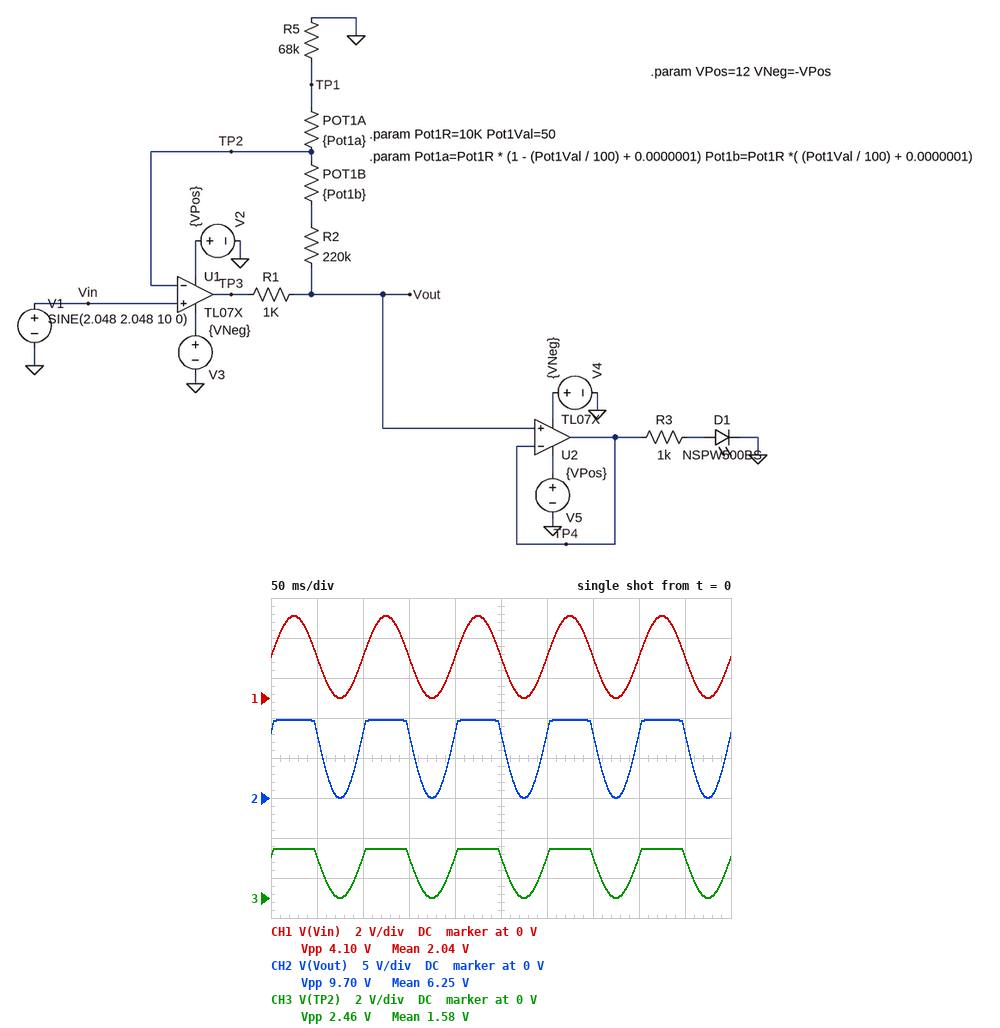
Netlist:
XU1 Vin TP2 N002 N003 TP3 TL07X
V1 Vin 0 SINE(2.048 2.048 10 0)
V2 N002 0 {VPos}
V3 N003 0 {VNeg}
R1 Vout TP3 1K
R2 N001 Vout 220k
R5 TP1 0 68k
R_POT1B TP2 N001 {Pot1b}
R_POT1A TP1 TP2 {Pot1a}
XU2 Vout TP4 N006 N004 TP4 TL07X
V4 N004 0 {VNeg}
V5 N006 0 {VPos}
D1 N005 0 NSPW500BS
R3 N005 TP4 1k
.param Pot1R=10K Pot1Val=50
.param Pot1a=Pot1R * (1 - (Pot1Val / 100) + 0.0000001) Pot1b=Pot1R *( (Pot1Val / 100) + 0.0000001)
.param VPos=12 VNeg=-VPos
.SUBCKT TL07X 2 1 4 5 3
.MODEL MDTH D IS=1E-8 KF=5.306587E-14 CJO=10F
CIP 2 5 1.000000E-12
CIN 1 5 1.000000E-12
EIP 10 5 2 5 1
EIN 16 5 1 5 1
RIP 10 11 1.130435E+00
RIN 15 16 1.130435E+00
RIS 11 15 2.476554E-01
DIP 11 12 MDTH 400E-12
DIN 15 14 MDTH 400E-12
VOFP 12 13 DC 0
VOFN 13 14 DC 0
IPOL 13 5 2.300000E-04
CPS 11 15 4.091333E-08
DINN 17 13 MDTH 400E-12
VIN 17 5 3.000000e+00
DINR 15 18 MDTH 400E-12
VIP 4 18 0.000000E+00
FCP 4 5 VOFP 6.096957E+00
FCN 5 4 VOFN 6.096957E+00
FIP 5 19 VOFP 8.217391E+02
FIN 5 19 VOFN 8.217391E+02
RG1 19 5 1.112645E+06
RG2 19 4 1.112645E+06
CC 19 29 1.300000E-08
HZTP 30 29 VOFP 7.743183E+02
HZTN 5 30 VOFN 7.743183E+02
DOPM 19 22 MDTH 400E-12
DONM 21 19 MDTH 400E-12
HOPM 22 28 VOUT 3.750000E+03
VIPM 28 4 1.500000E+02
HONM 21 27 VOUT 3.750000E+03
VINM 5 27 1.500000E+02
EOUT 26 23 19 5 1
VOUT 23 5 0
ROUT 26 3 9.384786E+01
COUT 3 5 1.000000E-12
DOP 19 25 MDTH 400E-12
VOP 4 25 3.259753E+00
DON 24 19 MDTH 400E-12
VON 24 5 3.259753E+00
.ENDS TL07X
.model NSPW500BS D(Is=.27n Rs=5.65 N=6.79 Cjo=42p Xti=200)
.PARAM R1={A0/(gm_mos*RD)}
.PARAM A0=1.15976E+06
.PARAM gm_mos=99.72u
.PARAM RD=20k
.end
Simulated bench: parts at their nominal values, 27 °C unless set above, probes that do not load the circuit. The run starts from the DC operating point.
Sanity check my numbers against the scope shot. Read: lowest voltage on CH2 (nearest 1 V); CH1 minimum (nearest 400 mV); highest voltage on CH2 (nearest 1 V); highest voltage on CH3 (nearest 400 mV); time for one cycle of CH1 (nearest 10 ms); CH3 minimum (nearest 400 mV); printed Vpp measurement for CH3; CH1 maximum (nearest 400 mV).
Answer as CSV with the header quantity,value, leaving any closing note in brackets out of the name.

quantity,value
lowest voltage on CH2,0 V
CH1 minimum,0 V
highest voltage on CH2,10 V
highest voltage on CH3,2.4 V
time for one cycle of CH1,100 ms
CH3 minimum,0 V
printed Vpp measurement for CH3,2.46 V
CH1 maximum,4.0 V
